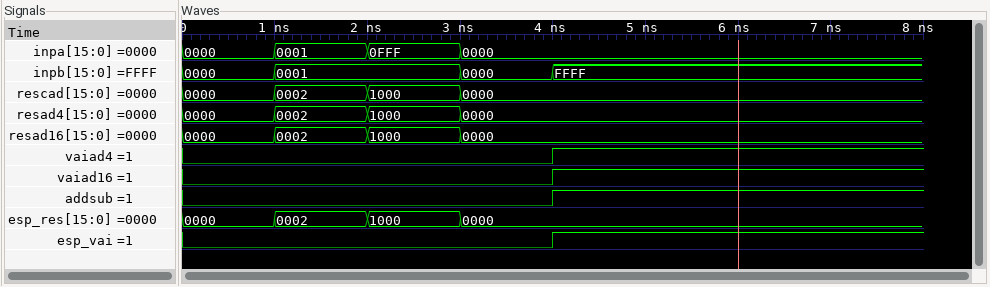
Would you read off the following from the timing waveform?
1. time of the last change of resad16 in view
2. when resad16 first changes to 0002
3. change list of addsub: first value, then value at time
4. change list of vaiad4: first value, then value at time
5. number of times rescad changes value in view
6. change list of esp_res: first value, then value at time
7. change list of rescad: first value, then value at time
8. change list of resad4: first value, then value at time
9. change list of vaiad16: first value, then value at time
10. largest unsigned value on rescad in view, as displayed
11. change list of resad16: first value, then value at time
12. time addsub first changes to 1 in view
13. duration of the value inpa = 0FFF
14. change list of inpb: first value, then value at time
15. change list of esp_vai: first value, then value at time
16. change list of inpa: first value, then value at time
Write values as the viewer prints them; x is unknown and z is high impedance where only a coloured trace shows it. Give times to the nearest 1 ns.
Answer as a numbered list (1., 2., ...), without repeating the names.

1. 3 ns
2. 1 ns
3. 0, 1 at 4 ns
4. 0, 1 at 4 ns
5. 3
6. 0000, 0002 at 1 ns, 1000 at 2 ns, 0000 at 3 ns
7. 0000, 0002 at 1 ns, 1000 at 2 ns, 0000 at 3 ns
8. 0000, 0002 at 1 ns, 1000 at 2 ns, 0000 at 3 ns
9. 0, 1 at 4 ns
10. 1000
11. 0000, 0002 at 1 ns, 1000 at 2 ns, 0000 at 3 ns
12. 4 ns
13. 1 ns
14. 0000, 0001 at 1 ns, 0000 at 3 ns, FFFF at 4 ns
15. 0, 1 at 4 ns
16. 0000, 0001 at 1 ns, 0FFF at 2 ns, 0000 at 3 ns
